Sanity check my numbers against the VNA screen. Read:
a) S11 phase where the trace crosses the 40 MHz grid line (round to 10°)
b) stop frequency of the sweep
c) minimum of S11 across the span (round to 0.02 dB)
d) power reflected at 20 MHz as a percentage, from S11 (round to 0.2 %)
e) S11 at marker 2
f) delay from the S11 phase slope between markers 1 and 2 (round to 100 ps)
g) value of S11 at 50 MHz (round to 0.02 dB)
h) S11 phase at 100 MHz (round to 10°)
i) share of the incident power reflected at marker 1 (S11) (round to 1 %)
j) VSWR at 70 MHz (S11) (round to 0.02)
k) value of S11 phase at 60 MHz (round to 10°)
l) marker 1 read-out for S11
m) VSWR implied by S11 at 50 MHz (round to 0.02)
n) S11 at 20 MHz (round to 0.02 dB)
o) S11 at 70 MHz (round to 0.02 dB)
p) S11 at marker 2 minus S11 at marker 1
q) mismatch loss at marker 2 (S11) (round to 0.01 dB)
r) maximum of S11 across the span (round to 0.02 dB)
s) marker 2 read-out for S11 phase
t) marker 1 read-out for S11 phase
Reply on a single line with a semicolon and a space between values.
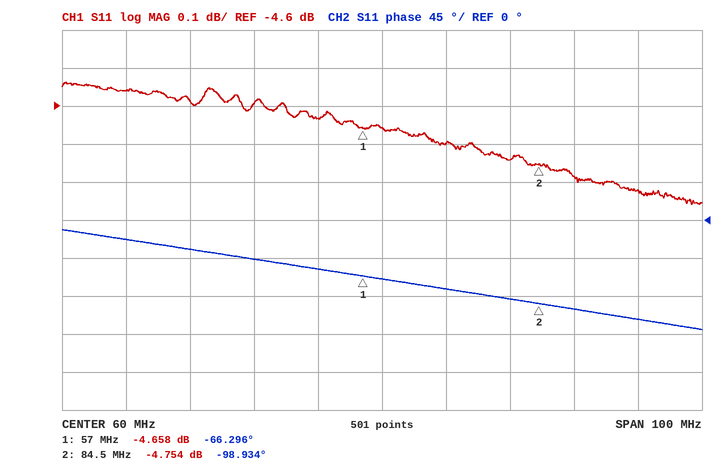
-50°; 110 MHz; -4.86 dB; 35.0 %; -4.754 dB; 3.3 ns; -4.64 dB; -120°; 34 %; 3.78; -70°; -4.658 dB; 3.84; -4.56 dB; -4.70 dB; -0.096 dB; 1.77 dB; -4.54 dB; -98.934°; -66.296°
